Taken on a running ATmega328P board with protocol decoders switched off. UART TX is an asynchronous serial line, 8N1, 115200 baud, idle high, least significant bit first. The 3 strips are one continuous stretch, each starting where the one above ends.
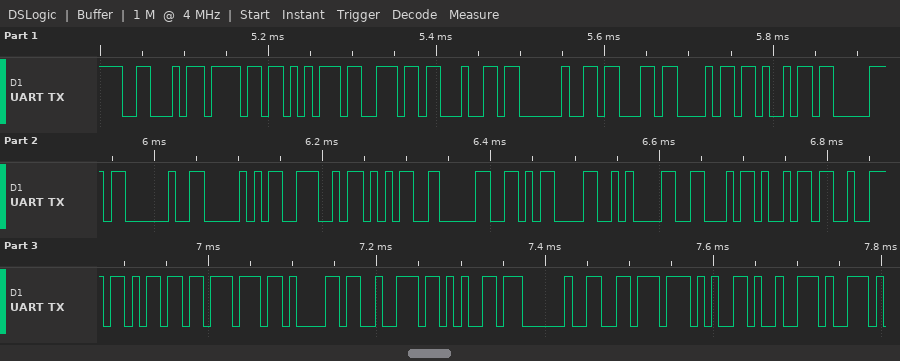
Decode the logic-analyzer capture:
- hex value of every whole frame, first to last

46 6F 75 6E 64 20 63 68 69 70 20 50 4E 35 30 0D 0A 46 69 72 6D 77 61 72 65 20 76 65 72
